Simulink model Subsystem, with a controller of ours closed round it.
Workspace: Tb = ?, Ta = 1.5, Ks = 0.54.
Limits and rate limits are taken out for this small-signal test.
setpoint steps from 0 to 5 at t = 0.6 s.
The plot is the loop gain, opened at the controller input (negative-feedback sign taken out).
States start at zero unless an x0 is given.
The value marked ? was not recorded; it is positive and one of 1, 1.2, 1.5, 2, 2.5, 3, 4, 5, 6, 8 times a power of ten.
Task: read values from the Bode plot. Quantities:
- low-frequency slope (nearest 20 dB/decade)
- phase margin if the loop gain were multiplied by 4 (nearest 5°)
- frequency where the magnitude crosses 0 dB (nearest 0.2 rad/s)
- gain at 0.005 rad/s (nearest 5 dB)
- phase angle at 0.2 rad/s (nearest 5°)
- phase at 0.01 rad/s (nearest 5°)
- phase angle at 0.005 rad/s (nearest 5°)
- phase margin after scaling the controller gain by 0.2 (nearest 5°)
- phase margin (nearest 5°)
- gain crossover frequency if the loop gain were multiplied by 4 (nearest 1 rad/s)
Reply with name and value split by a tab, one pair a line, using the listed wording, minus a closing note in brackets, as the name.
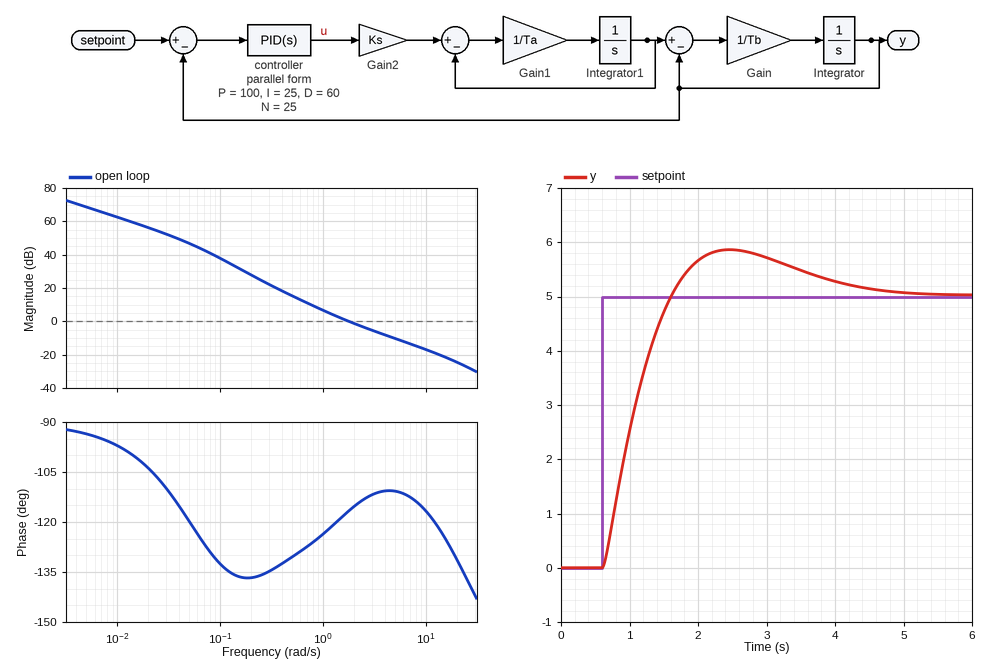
low-frequency slope	-20 dB/decade
phase margin if the loop gain were multiplied by 4	70°
frequency where the magnitude crosses 0 dB	1.8 rad/s
gain at 0.005 rad/s	70 dB
phase angle at 0.2 rad/s	-135°
phase at 0.01 rad/s	-95°
phase angle at 0.005 rad/s	-95°
phase margin after scaling the controller gain by 0.2	50°
phase margin	65°
gain crossover frequency if the loop gain were multiplied by 4	6 rad/s
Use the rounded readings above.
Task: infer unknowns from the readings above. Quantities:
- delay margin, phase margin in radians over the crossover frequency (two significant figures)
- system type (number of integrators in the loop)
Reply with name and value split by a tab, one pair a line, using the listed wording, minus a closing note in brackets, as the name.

delay margin, phase margin in radians over the crossover frequency	0.63 s
system type	1
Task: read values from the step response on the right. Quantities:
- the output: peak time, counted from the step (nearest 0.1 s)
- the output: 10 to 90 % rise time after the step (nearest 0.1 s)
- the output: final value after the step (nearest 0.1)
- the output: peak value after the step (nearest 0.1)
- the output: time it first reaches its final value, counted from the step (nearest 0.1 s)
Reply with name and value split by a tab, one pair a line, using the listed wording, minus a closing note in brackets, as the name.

the output: peak time, counted from the step	1.9 s
the output: 10 to 90 % rise time after the step	0.7 s
the output: final value after the step	5.0
the output: peak value after the step	5.9
the output: time it first reaches its final value, counted from the step	1.0 s
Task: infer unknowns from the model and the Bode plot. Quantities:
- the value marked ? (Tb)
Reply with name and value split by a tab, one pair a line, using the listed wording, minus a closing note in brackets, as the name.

the value marked ?	15
